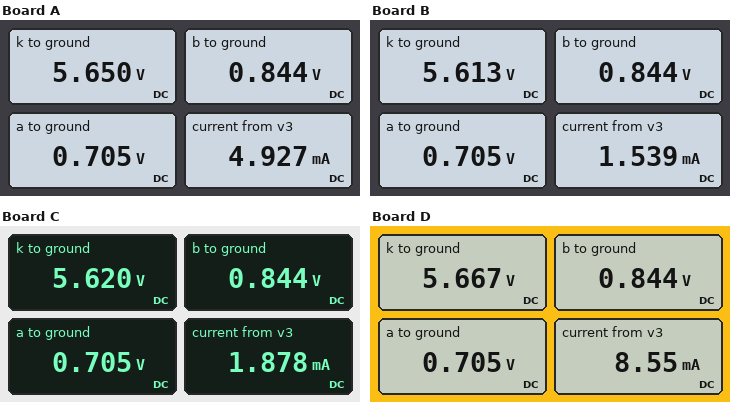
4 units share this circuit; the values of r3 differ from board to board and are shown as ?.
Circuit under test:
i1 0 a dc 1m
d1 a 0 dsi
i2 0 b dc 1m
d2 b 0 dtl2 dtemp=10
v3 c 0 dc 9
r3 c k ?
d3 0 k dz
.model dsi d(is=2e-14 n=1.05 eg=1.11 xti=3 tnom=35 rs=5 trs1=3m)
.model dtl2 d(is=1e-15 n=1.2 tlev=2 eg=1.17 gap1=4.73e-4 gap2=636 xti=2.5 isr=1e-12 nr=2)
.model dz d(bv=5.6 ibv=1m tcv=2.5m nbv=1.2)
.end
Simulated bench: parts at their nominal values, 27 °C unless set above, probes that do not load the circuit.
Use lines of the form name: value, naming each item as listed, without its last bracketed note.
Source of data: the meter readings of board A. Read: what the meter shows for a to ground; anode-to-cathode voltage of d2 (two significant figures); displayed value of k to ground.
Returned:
what the meter shows for a to ground: 0.705 V
anode-to-cathode voltage of d2: 840 mV
displayed value of k to ground: 5.650 V
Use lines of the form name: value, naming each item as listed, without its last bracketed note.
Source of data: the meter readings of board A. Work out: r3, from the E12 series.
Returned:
r3, from the E12 series: 680 Ω
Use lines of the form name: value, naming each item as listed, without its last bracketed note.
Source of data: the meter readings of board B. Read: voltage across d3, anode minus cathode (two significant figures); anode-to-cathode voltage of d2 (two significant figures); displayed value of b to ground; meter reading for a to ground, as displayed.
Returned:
voltage across d3, anode minus cathode: -5.6 V
anode-to-cathode voltage of d2: 840 mV
displayed value of b to ground: 0.844 V
meter reading for a to ground, as displayed: 0.705 V
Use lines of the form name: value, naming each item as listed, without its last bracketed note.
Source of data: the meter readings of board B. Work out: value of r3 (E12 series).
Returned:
value of r3: 2.2 kΩ
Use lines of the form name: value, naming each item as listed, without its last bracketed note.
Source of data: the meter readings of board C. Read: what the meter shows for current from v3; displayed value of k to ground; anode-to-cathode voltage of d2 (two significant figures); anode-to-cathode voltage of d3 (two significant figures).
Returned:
what the meter shows for current from v3: 1.878 mA
displayed value of k to ground: 5.620 V
anode-to-cathode voltage of d2: 840 mV
anode-to-cathode voltage of d3: -5.6 V
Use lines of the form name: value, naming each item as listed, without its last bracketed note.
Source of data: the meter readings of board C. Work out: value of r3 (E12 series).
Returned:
value of r3: 1.8 kΩ
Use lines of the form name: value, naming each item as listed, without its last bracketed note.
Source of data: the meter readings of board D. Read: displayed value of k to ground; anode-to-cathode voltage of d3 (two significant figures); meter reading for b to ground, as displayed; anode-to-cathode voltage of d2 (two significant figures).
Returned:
displayed value of k to ground: 5.667 V
anode-to-cathode voltage of d3: -5.7 V
meter reading for b to ground, as displayed: 0.844 V
anode-to-cathode voltage of d2: 840 mV
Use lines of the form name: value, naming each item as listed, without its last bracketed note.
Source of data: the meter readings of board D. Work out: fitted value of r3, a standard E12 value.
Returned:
fitted value of r3, a standard E12 value: 390 Ω
